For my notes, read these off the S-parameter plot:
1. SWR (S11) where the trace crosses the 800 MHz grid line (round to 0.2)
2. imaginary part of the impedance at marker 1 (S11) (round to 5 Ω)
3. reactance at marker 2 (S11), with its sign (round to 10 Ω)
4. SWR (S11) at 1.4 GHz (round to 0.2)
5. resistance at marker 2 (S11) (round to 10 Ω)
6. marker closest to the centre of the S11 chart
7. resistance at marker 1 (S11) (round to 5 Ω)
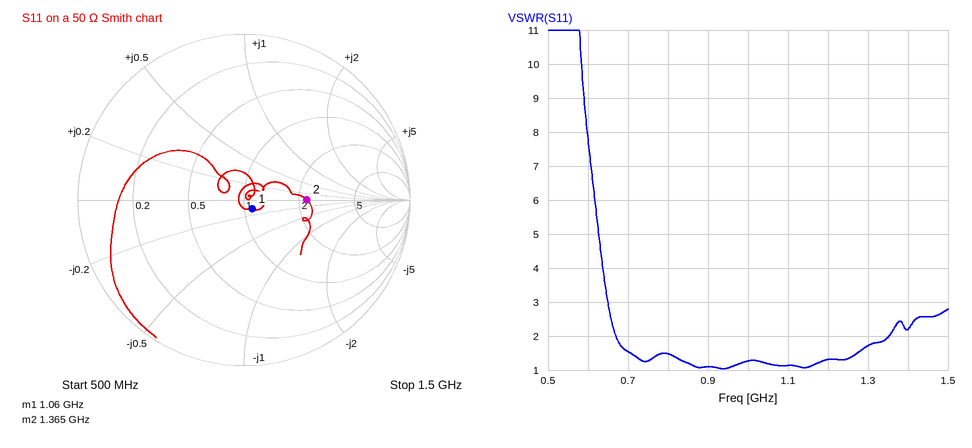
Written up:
1.4
-5 Ω
0 Ω
2.2
110 Ω
marker 1
55 Ω
